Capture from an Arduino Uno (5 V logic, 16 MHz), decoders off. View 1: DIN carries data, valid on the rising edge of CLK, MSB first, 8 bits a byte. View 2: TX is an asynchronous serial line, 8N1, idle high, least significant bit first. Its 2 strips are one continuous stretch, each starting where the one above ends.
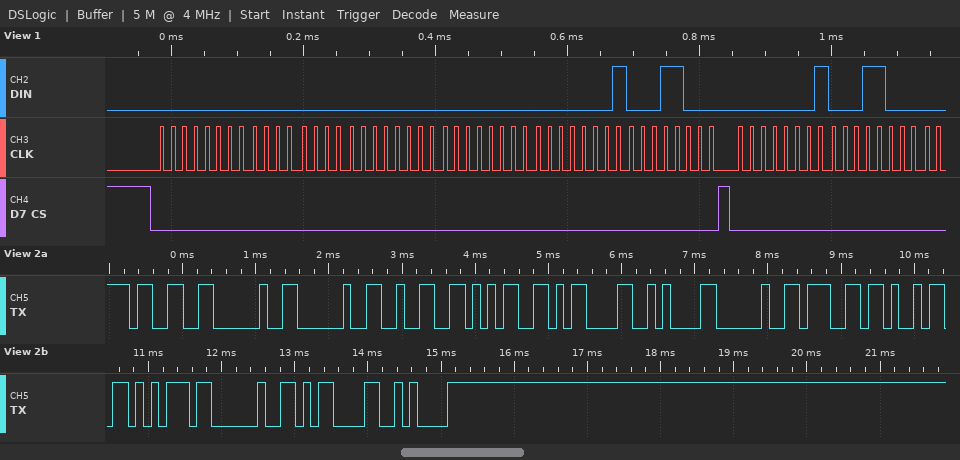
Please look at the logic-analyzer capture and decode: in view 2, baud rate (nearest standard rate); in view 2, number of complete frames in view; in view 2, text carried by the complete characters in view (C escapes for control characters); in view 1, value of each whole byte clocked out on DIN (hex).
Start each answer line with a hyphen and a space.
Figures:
- 9600 baud
- 14
- "3  25\r\n giu \r\n"
- 00 00 00 00 01 18 01 18
